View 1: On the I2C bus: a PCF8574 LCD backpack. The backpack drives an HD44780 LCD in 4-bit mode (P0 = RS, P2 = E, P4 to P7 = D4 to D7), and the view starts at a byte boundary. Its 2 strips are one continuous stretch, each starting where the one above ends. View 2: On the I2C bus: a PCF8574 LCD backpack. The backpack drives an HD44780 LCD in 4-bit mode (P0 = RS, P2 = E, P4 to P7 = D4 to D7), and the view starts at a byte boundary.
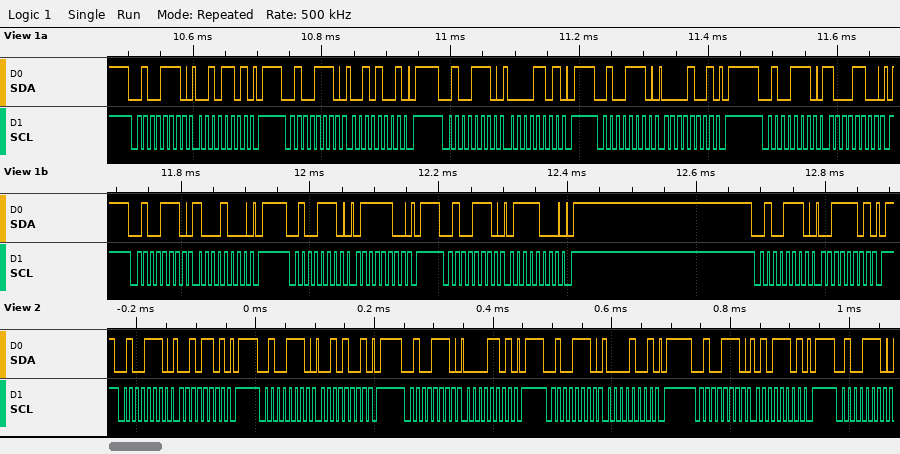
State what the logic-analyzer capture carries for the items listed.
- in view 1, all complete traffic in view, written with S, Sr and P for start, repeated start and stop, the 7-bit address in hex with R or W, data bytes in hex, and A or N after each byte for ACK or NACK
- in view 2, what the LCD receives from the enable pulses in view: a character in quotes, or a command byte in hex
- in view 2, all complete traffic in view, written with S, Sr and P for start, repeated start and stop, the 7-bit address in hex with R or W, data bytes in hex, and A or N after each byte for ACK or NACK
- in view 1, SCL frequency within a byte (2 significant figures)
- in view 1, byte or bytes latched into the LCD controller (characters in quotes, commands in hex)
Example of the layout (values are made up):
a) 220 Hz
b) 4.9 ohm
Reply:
a) S 27W A 2D A P S 27W A 29 A P S 27W A 0D A P S 27W A 09 A P S 27W A 8C A P S 27W A 88 A P S 27W A 7C A P S 27W A 78 A P S 27W A 3D A P
b) ' '
c) S 27W A 2D A P S 27W A 29 A P S 27W A 0D A P S 27W A 09 A P S 27W A 5D A P S 27W A
d) 100 kHz
e) ' ' 0x87
